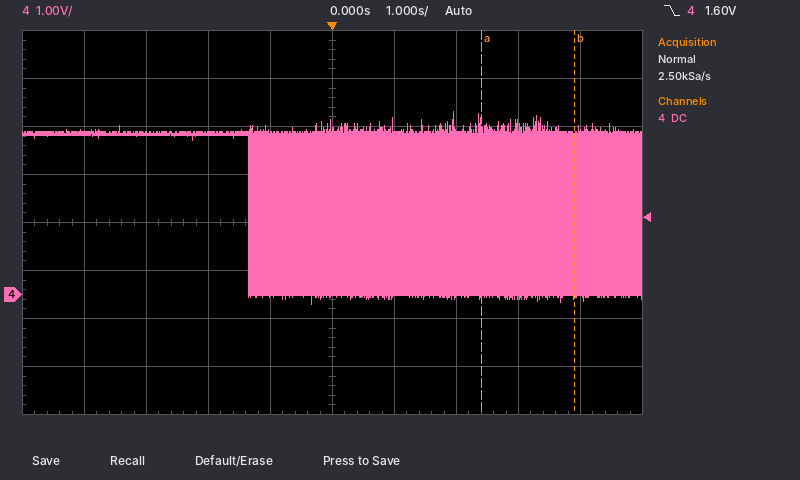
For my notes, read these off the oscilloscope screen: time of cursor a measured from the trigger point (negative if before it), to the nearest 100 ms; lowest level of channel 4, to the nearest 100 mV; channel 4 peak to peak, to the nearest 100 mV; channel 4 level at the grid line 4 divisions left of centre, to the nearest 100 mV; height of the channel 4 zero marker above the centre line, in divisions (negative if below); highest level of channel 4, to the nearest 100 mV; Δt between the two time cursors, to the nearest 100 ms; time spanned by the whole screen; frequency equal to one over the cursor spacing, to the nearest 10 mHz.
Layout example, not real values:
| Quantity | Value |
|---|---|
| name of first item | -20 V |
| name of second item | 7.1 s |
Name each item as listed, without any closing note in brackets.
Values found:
| Quantity | Value |
|---|---|
| time of cursor a measured from the trigger point (negative if before it), to the nearest 100 ms | +2.4 s |
| lowest level of channel 4, to the nearest 100 mV | -200 mV |
| channel 4 peak to peak, to the nearest 100 mV | 4.0 V |
| channel 4 level at the grid line 4 divisions left of centre, to the nearest 100 mV | 3.4 V |
| height of the channel 4 zero marker above the centre line, in divisions | -1.5 div |
| highest level of channel 4, to the nearest 100 mV | 3.8 V |
| Δt between the two time cursors, to the nearest 100 ms | 1.5 s |
| time spanned by the whole screen | 10 s |
| frequency equal to one over the cursor spacing, to the nearest 10 mHz | 670 mHz |
